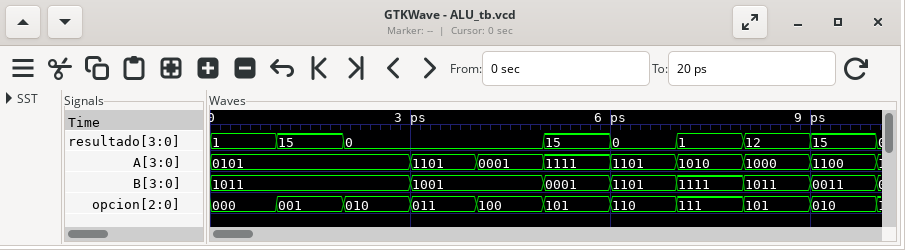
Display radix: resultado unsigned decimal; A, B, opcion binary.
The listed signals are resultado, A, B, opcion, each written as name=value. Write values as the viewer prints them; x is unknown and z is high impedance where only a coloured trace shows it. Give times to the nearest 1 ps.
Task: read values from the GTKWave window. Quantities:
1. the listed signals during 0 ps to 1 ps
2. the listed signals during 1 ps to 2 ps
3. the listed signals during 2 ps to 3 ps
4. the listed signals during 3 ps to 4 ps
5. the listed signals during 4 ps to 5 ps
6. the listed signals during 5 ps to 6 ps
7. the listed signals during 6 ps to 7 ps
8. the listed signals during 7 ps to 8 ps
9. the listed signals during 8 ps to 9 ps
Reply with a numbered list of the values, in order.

1. resultado=1, A=0101, B=1011, opcion=000
2. resultado=15, A=0101, B=1011, opcion=001
3. resultado=0, A=0101, B=1011, opcion=010
4. resultado=0, A=1101, B=1001, opcion=011
5. resultado=0, A=0001, B=1001, opcion=100
6. resultado=15, A=1111, B=0001, opcion=101
7. resultado=0, A=1101, B=1101, opcion=110
8. resultado=1, A=1010, B=1111, opcion=111
9. resultado=12, A=1000, B=1011, opcion=101
